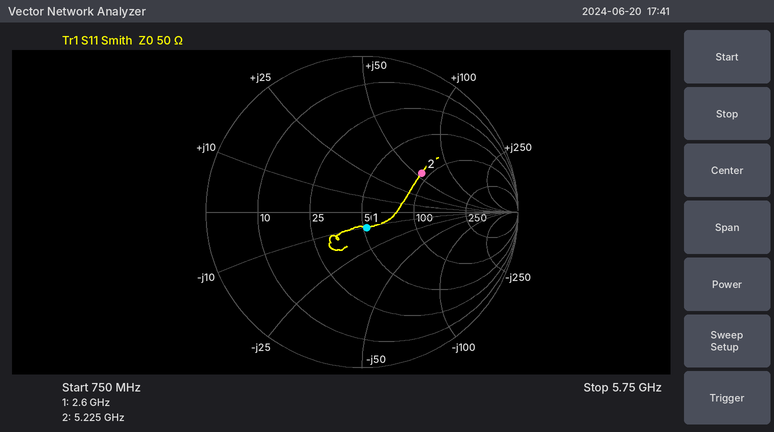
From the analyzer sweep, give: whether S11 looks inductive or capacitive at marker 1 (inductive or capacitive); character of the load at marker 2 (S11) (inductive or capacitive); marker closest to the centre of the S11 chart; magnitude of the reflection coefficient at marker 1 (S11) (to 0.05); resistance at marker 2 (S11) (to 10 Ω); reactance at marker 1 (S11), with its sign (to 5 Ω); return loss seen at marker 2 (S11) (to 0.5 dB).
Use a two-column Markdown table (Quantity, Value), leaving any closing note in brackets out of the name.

| Quantity | Value |
|---|---|
| whether S11 looks inductive or capacitive at marker 1 | capacitive |
| character of the load at marker 2 (S11) | inductive |
| marker closest to the centre of the S11 chart | marker 1 |
| magnitude of the reflection coefficient at marker 1 (S11) | 0.10 |
| resistance at marker 2 (S11) | 90 Ω |
| reactance at marker 1 (S11), with its sign | -10 Ω |
| return loss seen at marker 2 (S11) | 7.0 dB |
